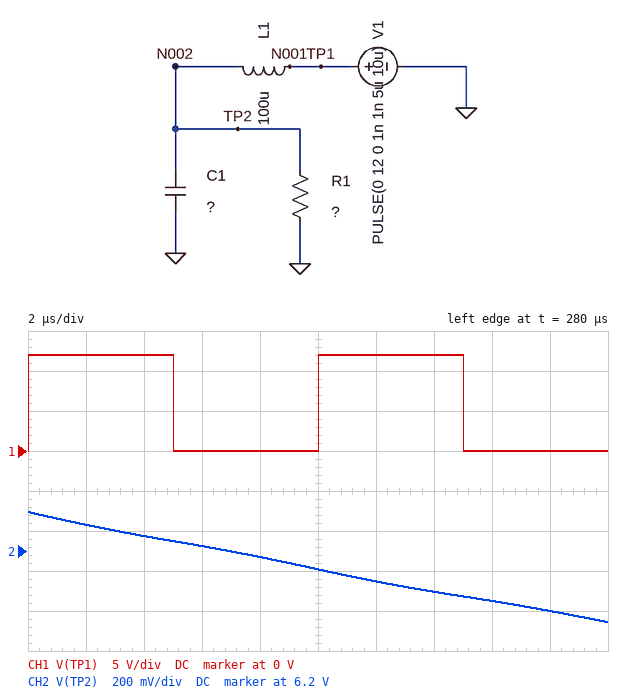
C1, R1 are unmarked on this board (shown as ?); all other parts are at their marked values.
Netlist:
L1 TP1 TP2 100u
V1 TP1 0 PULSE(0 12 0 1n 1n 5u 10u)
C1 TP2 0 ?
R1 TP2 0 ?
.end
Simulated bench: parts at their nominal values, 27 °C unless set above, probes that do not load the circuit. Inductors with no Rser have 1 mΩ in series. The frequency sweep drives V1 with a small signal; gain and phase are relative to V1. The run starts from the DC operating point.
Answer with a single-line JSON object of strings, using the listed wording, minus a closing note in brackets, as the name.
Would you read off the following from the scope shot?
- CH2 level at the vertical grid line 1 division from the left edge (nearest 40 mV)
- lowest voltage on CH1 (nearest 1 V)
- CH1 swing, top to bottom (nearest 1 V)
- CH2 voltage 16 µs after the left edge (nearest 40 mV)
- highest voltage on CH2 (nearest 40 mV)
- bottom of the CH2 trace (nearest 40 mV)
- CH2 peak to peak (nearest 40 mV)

{"CH2 level at the vertical grid line 1 division from the left edge": "6.32 V", "lowest voltage on CH1": "0 V", "CH1 swing, top to bottom": "12 V", "CH2 voltage 16 µs after the left edge": "5.96 V", "highest voltage on CH2": "6.40 V", "bottom of the CH2 trace": "5.84 V", "CH2 peak to peak": "560 mV"}
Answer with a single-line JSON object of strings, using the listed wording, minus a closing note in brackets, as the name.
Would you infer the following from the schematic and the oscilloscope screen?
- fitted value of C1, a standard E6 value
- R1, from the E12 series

{"fitted value of C1, a standard E6 value": "33 µF", "R1, from the E12 series": "3.3 Ω"}
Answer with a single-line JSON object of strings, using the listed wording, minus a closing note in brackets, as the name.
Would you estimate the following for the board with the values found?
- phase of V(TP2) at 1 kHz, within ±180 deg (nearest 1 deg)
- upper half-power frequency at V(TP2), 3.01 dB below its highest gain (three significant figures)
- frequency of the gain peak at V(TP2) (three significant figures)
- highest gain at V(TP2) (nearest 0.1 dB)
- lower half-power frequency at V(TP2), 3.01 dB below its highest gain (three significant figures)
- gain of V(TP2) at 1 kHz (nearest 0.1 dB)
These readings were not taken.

{"phase of V(TP2) at 1 kHz, within ±180 deg": "-12 deg", "upper half-power frequency at V(TP2), 3.01 dB below its highest gain": "3.24 kHz", "frequency of the gain peak at V(TP2)": "2.57 kHz", "highest gain at V(TP2)": "5.9 dB", "lower half-power frequency at V(TP2), 3.01 dB below its highest gain": "1.64 kHz", "gain of V(TP2) at 1 kHz": "1.0 dB"}
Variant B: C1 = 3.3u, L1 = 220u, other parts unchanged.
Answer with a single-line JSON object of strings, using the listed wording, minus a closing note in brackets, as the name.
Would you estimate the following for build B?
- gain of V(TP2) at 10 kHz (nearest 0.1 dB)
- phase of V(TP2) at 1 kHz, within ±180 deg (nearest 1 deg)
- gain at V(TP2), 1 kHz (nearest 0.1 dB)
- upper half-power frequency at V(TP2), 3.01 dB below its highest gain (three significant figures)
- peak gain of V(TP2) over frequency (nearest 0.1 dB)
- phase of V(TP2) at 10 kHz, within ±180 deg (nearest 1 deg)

{"gain of V(TP2) at 10 kHz": "-13.2 dB", "phase of V(TP2) at 1 kHz, within ±180 deg": "-23 deg", "gain at V(TP2), 1 kHz": "-0.5 dB", "upper half-power frequency at V(TP2), 3.01 dB below its highest gain": "2.83 kHz", "peak gain of V(TP2) over frequency": "0 dB", "phase of V(TP2) at 10 kHz, within ±180 deg": "-114 deg"}
